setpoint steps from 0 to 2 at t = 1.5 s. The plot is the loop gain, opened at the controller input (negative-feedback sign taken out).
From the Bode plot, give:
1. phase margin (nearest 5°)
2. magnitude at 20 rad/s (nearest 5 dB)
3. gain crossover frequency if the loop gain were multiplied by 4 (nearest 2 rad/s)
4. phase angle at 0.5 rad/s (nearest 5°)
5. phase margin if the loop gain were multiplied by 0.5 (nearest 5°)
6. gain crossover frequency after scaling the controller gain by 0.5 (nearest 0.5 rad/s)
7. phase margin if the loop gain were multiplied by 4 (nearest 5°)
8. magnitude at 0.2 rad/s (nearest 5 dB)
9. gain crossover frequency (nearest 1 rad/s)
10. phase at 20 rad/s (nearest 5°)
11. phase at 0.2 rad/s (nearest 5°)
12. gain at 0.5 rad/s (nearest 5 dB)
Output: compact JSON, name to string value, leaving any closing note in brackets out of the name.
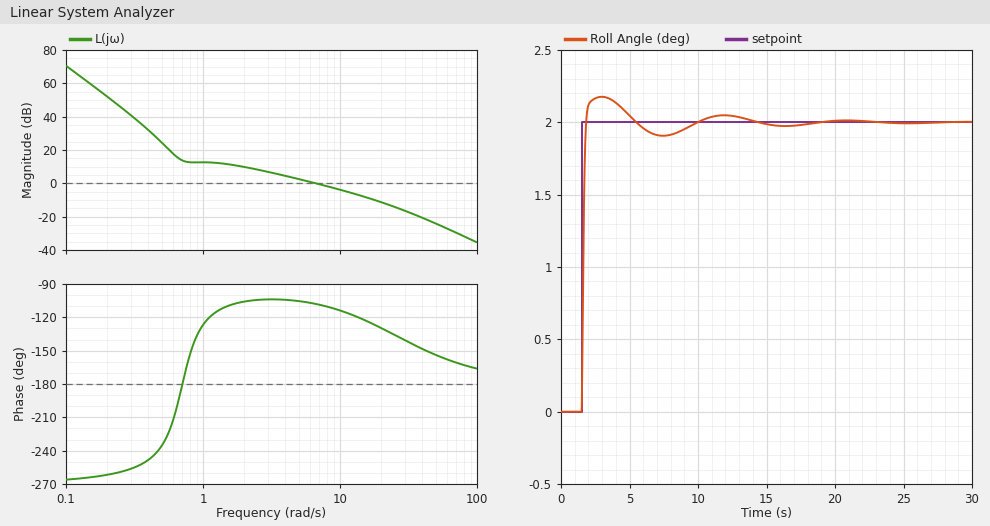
{"phase margin": "70°", "magnitude at 20 rad/s": "-10 dB", "gain crossover frequency if the loop gain were multiplied by 4": "22 rad/s", "phase angle at 0.5 rad/s": "-235°", "phase margin if the loop gain were multiplied by 0.5": "75°", "gain crossover frequency after scaling the controller gain by 0.5": "3.5 rad/s", "phase margin if the loop gain were multiplied by 4": "50°", "magnitude at 0.2 rad/s": "50 dB", "gain crossover frequency": "7 rad/s", "phase at 20 rad/s": "-130°", "phase at 0.2 rad/s": "-260°", "gain at 0.5 rad/s": "25 dB"}
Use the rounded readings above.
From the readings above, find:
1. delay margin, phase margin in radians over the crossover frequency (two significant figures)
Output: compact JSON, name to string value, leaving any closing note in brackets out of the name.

{"delay margin, phase margin in radians over the crossover frequency": "0.17 s"}
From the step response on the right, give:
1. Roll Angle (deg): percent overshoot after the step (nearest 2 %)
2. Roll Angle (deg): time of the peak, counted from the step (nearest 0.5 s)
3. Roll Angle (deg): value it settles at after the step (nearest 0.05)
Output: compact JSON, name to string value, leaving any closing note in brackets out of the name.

{"Roll Angle (deg): percent overshoot after the step": "8 %", "Roll Angle (deg): time of the peak, counted from the step": "1.5 s", "Roll Angle (deg): value it settles at after the step": "2.00"}
